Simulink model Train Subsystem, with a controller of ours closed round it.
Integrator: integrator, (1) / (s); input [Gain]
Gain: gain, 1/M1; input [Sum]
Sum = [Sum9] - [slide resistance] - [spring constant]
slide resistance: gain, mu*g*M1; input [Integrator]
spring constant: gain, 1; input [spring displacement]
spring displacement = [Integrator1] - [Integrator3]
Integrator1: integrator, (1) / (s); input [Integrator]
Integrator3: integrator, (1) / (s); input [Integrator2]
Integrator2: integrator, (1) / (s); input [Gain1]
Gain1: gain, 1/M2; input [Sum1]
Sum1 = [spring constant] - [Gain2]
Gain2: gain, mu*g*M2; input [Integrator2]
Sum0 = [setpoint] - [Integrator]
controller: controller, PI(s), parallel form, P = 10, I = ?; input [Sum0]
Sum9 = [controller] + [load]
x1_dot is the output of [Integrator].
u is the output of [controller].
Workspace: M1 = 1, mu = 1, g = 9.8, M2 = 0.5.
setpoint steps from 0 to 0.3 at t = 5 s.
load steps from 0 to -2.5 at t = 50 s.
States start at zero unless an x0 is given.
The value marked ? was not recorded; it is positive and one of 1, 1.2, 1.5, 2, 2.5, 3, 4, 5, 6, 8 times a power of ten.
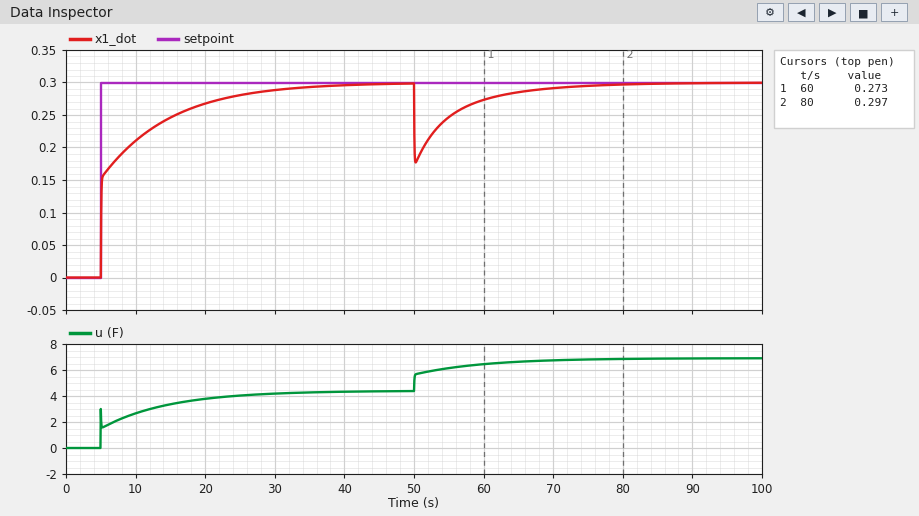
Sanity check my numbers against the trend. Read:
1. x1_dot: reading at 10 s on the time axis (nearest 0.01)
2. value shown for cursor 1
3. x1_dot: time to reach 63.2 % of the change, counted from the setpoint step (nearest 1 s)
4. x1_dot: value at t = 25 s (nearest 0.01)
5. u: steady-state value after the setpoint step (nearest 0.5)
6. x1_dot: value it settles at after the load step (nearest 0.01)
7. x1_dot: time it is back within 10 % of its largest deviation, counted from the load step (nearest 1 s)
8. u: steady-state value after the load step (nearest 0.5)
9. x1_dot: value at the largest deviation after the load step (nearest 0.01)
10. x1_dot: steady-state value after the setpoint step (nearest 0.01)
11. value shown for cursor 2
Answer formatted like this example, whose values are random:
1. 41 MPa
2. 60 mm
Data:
1. 0.21
2. 0.273
3. 3 s
4. 0.28
5. 4.5
6. 0.30
7. 17 s
8. 7.0
9. 0.18
10. 0.30
11. 0.297
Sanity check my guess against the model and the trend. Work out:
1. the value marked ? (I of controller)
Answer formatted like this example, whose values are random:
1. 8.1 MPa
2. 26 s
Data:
1. 3
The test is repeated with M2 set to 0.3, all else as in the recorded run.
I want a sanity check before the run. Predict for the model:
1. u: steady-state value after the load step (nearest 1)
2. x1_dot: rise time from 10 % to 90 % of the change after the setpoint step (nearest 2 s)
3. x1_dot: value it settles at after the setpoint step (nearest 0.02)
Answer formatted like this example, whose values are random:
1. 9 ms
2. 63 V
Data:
1. 6
2. 14 s
3. 0.30
